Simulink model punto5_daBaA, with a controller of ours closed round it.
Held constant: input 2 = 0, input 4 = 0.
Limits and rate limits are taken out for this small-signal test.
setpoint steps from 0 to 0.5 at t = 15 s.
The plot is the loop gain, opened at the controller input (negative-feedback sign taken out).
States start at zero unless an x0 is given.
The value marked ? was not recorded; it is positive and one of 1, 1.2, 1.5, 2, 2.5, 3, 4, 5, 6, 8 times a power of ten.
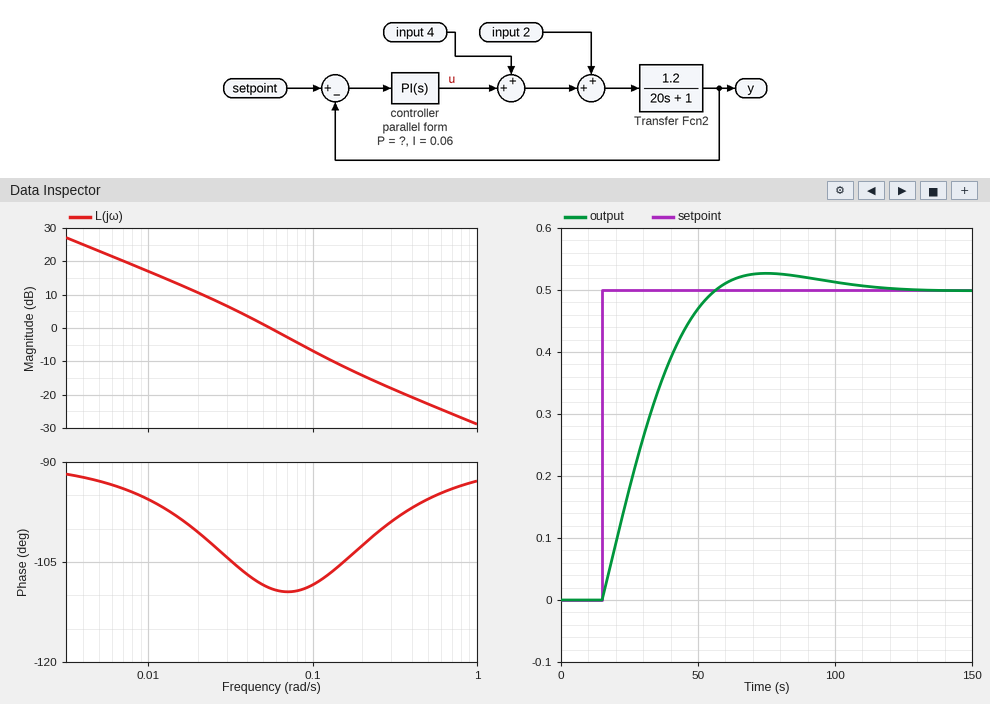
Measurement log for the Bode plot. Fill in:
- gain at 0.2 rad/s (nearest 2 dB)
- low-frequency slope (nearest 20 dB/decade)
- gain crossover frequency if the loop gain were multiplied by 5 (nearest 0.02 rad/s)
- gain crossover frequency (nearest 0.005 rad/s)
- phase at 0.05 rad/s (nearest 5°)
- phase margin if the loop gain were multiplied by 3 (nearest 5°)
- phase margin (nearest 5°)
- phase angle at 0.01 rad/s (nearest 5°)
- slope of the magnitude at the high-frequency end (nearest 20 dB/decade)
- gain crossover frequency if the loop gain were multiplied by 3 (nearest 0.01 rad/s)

-14 dB
-20 dB/decade
0.20 rad/s
0.055 rad/s
-110°
75°
70°
-95°
-20 dB/decade
0.13 rad/s
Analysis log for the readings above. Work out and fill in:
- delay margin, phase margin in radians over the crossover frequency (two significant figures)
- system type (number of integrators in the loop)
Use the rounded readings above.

22 s
1
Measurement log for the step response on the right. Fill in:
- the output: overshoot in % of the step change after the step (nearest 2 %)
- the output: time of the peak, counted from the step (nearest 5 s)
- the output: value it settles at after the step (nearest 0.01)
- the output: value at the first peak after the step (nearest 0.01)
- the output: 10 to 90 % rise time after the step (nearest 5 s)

6 %
60 s
0.50
0.53
30 s
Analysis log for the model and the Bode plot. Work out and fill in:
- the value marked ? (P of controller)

0.6
